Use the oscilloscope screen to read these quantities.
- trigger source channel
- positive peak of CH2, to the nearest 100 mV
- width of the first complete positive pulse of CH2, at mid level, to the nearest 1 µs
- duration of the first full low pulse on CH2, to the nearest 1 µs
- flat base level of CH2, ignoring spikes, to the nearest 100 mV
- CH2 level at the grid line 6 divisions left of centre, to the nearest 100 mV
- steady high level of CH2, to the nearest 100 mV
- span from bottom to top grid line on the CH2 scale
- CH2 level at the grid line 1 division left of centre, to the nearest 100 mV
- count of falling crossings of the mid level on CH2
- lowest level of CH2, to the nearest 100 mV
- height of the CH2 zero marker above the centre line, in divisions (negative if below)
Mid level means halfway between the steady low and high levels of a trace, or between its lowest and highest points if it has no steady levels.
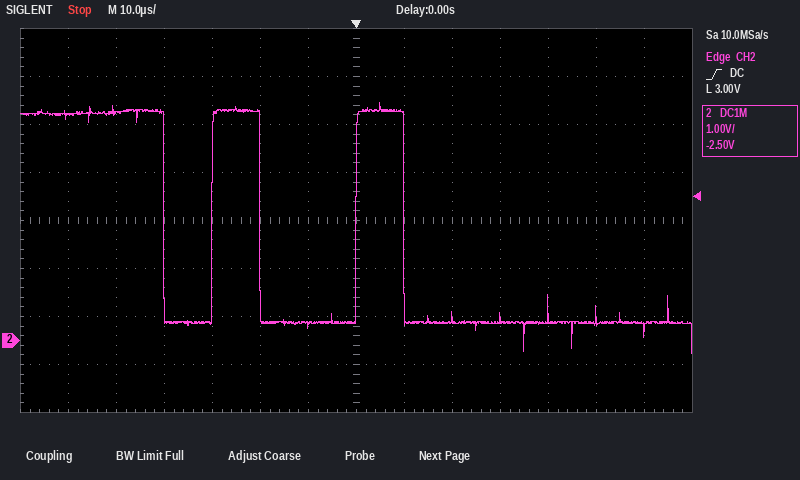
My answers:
CH2
5.0 V
10 µs
10 µs
400 mV
4.7 V
4.8 V
8 V
300 mV
3
-300 mV
-2.5 div
